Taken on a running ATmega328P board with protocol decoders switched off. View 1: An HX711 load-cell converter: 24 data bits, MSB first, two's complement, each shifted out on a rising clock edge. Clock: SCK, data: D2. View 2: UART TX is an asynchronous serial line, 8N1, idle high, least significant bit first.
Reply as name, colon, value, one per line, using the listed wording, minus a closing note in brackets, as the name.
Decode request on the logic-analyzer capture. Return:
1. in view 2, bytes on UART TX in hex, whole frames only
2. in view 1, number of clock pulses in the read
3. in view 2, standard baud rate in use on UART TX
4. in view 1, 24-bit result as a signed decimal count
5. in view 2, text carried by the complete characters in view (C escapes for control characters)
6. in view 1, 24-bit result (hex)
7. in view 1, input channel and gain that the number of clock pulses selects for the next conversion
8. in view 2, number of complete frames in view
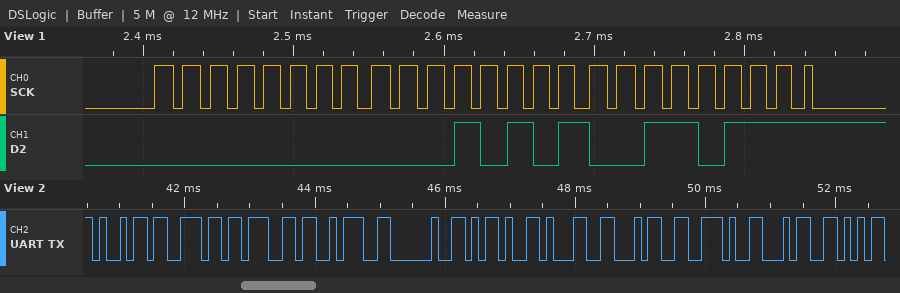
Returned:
in view 2, bytes on UART TX in hex, whole frames only: 69 6E 67 3A 20 2D 31 34 2E 34
in view 1, number of clock pulses in the read: 25
in view 2, standard baud rate in use on UART TX: 9600 baud
in view 1, 24-bit result as a signed decimal count: 5431
in view 2, text carried by the complete characters in view: "ing: -14.4"
in view 1, 24-bit result: 0x001537
in view 1, input channel and gain that the number of clock pulses selects for the next conversion: channel A, gain 128
in view 2, number of complete frames in view: 10
